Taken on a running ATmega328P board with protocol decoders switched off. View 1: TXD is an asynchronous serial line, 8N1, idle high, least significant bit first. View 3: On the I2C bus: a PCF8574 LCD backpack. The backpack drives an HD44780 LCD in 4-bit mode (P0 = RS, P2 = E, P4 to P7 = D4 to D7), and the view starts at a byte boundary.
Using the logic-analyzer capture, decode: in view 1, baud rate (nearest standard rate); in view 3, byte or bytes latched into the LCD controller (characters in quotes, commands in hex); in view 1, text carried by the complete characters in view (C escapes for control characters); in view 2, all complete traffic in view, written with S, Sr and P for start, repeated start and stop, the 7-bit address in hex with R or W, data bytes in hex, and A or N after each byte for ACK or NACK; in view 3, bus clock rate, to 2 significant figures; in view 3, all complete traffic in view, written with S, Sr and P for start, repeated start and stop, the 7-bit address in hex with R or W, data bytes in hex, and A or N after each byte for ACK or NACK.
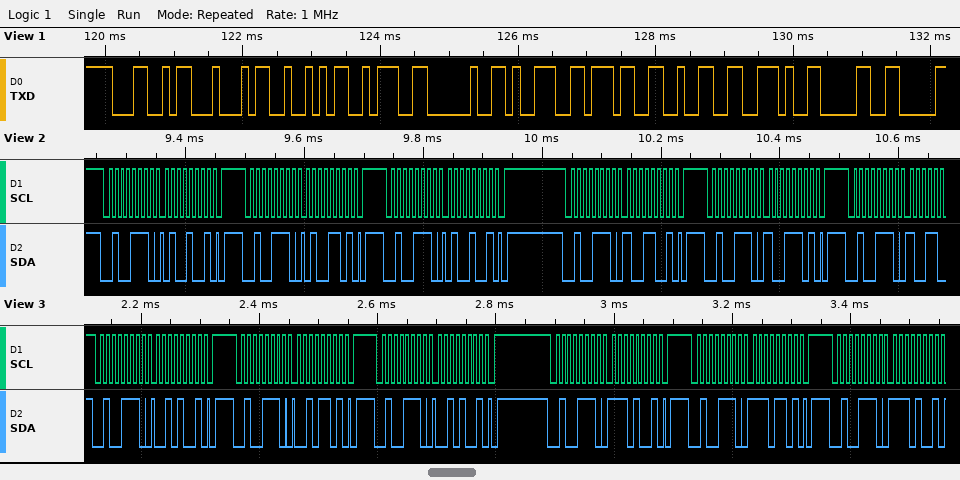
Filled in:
9600 baud
'.'
"LDR: 972.0"
S 27W A 49 A P S 27W A 4D A P S 27W A 49 A P S 27W A 99 A P S 27W A 9D A P S 27W A
100 kHz
S 27W A 29 A P S 27W A 2D A P S 27W A 29 A P S 27W A E9 A P S 27W A ED A P S 27W A E9 A
